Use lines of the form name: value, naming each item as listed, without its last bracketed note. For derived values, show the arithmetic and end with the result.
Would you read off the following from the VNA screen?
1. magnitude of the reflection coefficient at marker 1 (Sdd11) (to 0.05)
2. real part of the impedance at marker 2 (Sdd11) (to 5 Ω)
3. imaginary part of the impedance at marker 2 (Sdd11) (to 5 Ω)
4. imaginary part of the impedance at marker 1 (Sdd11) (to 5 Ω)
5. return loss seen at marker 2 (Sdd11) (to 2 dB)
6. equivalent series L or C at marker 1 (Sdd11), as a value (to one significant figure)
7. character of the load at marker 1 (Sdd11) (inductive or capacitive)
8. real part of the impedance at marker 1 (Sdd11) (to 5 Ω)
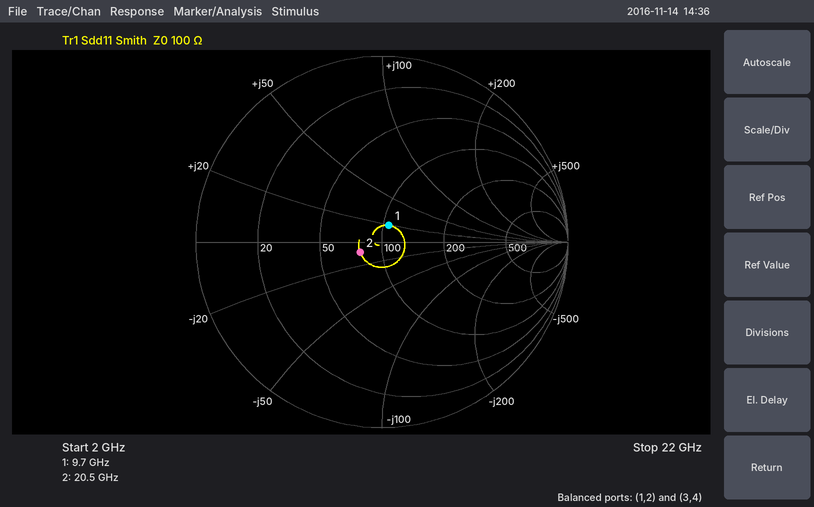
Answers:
magnitude of the reflection coefficient at marker 1 (Sdd11): 0.10
real part of the impedance at marker 2 (Sdd11): 80 Ω
imaginary part of the impedance at marker 2 (Sdd11): -10 Ω
imaginary part of the impedance at marker 1 (Sdd11): +20 Ω
return loss seen at marker 2 (Sdd11): 18 dB
equivalent series L or C at marker 1 (Sdd11), as a value: L = 20 Ω/(2π × 9.7 GHz) ≈ 328 pH, so 300 pH to one significant figure
character of the load at marker 1 (Sdd11): inductive
real part of the impedance at marker 1 (Sdd11): 105 Ω
